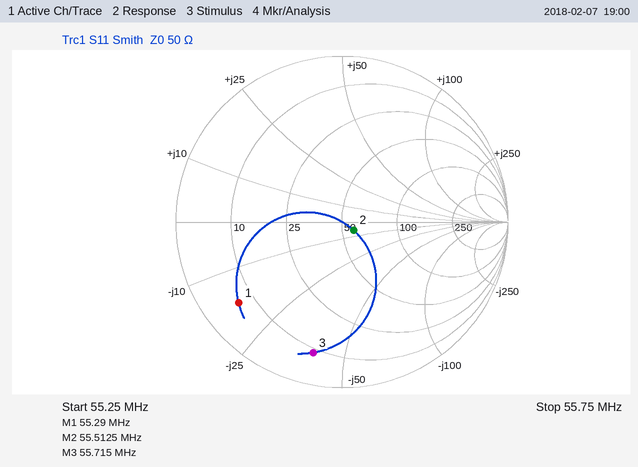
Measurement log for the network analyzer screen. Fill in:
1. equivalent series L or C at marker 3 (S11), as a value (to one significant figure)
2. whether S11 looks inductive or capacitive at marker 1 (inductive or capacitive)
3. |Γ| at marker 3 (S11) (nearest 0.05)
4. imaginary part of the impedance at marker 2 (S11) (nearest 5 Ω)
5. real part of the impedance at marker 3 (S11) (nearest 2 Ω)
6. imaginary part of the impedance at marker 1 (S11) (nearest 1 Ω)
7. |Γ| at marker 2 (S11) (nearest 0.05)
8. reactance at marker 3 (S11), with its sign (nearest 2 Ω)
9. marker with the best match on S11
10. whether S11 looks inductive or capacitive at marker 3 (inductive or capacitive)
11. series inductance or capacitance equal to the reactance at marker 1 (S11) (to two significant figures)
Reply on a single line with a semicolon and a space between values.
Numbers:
70 pF; capacitive; 0.80; -5 Ω; 8 Ω; -17 Ω; 0.10; -40 Ω; marker 2; capacitive; 170 pF
